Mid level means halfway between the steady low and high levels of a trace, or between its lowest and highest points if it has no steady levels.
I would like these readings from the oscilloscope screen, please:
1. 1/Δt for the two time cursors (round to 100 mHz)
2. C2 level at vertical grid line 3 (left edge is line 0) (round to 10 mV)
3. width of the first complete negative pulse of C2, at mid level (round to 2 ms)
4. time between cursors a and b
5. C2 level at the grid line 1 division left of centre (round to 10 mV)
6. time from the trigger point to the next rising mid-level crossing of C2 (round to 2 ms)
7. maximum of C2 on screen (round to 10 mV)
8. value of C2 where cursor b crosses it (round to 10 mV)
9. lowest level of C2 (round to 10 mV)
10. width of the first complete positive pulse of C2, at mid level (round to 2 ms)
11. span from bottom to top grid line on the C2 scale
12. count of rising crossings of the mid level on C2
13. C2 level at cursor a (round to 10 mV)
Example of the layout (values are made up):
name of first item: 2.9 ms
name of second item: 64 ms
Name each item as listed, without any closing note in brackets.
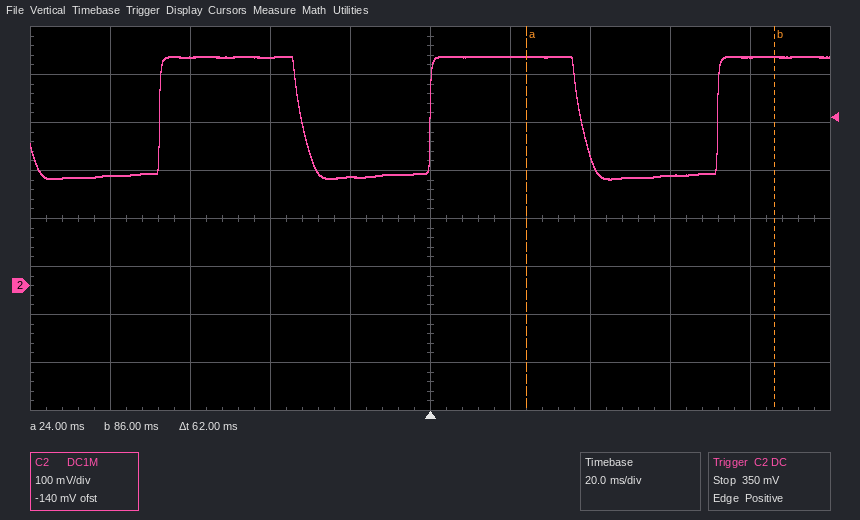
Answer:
1/Δt for the two time cursors: 16.1 Hz
C2 level at vertical grid line 3 (left edge is line 0): 480 mV
width of the first complete negative pulse of C2, at mid level: 32 ms
time between cursors a and b: 62 ms
C2 level at the grid line 1 division left of centre: 230 mV
time from the trigger point to the next rising mid-level crossing of C2: 72 ms
maximum of C2 on screen: 480 mV
value of C2 where cursor b crosses it: 480 mV
lowest level of C2: 220 mV
width of the first complete positive pulse of C2, at mid level: 36 ms
span from bottom to top grid line on the C2 scale: 800 mV
count of rising crossings of the mid level on C2: 3
C2 level at cursor a: 480 mV
